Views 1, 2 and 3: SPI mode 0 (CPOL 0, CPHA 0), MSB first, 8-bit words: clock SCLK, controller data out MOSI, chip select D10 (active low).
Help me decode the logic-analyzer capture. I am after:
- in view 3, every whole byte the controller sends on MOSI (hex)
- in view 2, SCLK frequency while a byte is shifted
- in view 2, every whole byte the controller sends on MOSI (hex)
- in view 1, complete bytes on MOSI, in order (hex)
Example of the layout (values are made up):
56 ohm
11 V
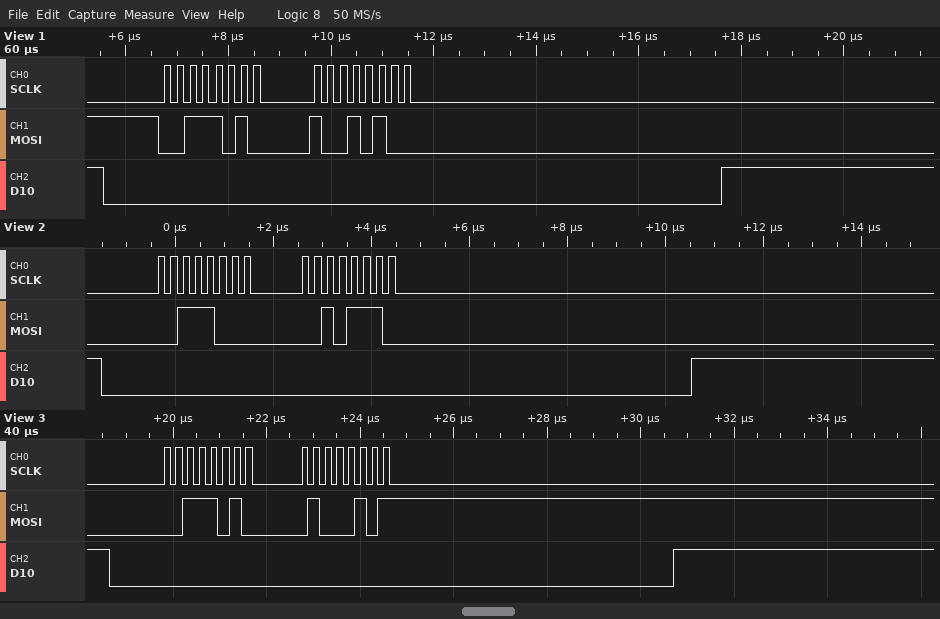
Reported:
0x3A 0x45
4 MHz
0x38 0x2E
3A 94
